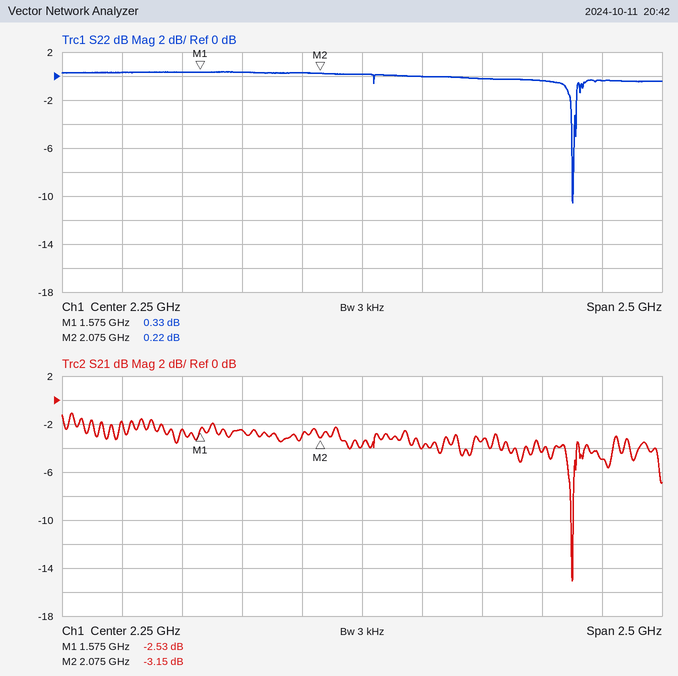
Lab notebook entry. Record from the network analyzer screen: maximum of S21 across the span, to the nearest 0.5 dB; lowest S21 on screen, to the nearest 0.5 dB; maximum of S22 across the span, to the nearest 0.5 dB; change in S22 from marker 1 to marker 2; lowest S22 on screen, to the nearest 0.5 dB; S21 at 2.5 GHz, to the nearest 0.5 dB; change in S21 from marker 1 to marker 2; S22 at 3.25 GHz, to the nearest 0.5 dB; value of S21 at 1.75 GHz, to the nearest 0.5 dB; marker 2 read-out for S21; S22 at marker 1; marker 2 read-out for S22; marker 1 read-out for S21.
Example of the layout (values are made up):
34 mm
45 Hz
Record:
-1.0 dB
-15.0 dB
0.5 dB
-0.11 dB
-10.5 dB
-4.0 dB
-0.62 dB
-0.5 dB
-2.5 dB
-3.15 dB
0.33 dB
0.22 dB
-2.53 dB
